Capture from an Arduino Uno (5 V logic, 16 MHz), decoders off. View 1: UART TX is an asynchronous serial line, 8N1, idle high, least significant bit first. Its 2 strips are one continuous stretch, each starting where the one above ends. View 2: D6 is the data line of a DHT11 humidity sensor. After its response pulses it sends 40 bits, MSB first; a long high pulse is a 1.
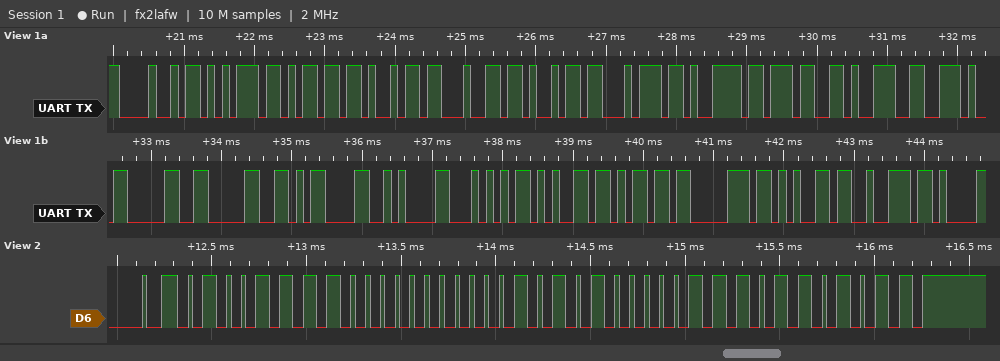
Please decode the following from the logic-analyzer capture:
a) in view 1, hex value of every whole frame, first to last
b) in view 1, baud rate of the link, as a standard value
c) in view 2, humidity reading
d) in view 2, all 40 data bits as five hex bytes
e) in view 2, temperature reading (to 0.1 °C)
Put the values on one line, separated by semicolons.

48 75 6D 69 64 69 74 79 37 39 2E 30 30 0D 0A 54 65 6D 70 65 72; 9600 baud; 79 %; 4F 00 15 07 6B; 21.7 °C
